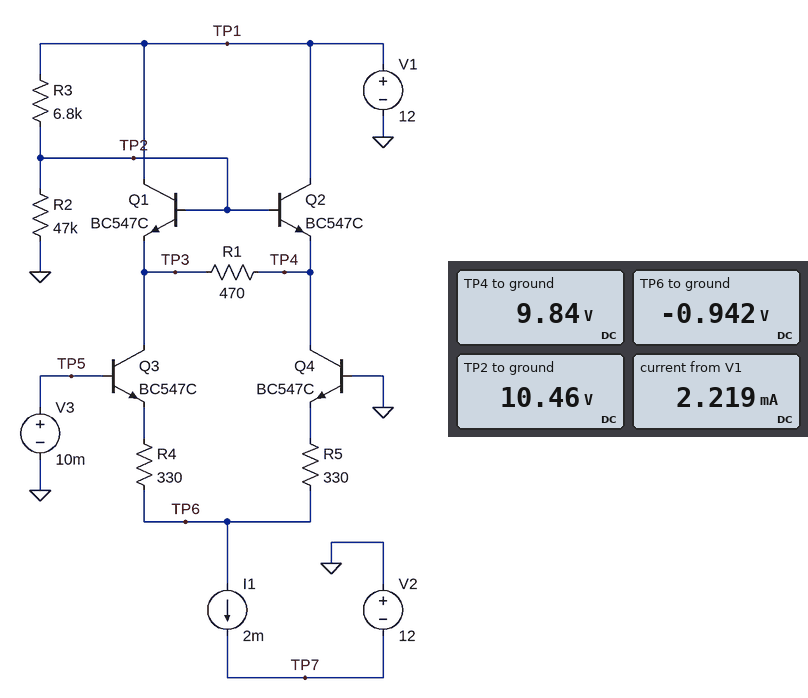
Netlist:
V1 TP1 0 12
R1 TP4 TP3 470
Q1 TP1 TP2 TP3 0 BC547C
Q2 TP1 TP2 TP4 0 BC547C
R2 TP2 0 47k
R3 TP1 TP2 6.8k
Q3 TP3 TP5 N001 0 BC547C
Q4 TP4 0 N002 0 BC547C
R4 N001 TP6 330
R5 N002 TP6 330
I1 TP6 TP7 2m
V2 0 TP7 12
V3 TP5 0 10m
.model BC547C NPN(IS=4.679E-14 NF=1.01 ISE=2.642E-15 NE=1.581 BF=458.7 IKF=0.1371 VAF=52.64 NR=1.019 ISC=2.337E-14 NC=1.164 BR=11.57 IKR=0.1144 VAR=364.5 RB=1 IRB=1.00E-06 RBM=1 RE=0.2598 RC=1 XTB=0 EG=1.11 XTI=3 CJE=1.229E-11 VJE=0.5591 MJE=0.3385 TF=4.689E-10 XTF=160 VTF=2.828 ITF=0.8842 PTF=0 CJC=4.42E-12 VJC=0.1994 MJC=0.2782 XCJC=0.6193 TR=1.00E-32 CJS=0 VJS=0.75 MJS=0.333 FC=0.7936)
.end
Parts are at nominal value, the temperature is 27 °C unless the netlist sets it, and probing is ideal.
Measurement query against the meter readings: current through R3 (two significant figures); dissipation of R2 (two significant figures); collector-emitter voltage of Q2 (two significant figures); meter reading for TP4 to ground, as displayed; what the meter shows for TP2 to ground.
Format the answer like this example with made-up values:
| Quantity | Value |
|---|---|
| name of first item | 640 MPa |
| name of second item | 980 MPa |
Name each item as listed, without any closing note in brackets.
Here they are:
| Quantity | Value |
|---|---|
| current through R3 | 230 µA |
| dissipation of R2 | 2.3 mW |
| collector-emitter voltage of Q2 | 2.2 V |
| meter reading for TP4 to ground, as displayed | 9.84 V |
| what the meter shows for TP2 to ground | 10.46 V |
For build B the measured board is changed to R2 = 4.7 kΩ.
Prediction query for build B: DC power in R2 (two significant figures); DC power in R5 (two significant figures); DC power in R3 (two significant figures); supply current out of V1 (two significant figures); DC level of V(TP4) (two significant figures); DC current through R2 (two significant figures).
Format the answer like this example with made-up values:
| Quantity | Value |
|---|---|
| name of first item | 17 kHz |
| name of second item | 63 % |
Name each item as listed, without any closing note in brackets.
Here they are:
| Quantity | Value |
|---|---|
| DC power in R2 | 5.1 mW |
| DC power in R5 | 320 µW |
| DC power in R3 | 7.4 mW |
| supply current out of V1 | 3.0 mA |
| DC level of V(TP4) | 4.3 V |
| DC current through R2 | 1.0 mA |
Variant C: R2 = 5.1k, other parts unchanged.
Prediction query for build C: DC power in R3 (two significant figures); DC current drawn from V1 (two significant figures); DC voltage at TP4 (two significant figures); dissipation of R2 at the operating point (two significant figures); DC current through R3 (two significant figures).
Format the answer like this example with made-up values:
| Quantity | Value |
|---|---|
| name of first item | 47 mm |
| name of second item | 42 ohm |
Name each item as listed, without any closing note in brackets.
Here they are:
| Quantity | Value |
|---|---|
| DC power in R3 | 6.9 mW |
| DC current drawn from V1 | 3.0 mA |
| DC voltage at TP4 | 4.5 V |
| dissipation of R2 at the operating point | 5.2 mW |
| DC current through R3 | 1.0 mA |
